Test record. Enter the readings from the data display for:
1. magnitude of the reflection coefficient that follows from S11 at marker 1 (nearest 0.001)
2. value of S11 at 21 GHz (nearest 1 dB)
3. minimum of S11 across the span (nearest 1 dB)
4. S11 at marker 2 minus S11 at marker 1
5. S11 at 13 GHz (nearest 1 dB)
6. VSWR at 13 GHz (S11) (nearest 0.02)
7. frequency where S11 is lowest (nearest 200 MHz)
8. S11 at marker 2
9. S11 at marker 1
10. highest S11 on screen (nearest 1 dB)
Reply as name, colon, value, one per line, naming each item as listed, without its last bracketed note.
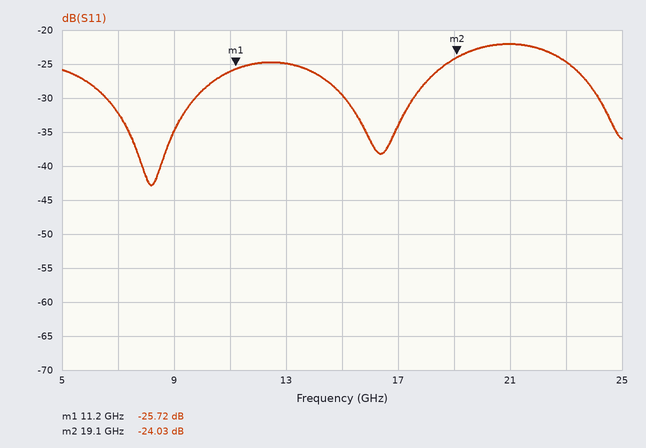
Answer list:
magnitude of the reflection coefficient that follows from S11 at marker 1: 0.052
value of S11 at 21 GHz: -22 dB
minimum of S11 across the span: -43 dB
S11 at marker 2 minus S11 at marker 1: 1.69 dB
S11 at 13 GHz: -25 dB
VSWR at 13 GHz (S11): 1.12
frequency where S11 is lowest: 8.2 GHz
S11 at marker 2: -24.03 dB
S11 at marker 1: -25.72 dB
highest S11 on screen: -22 dB
